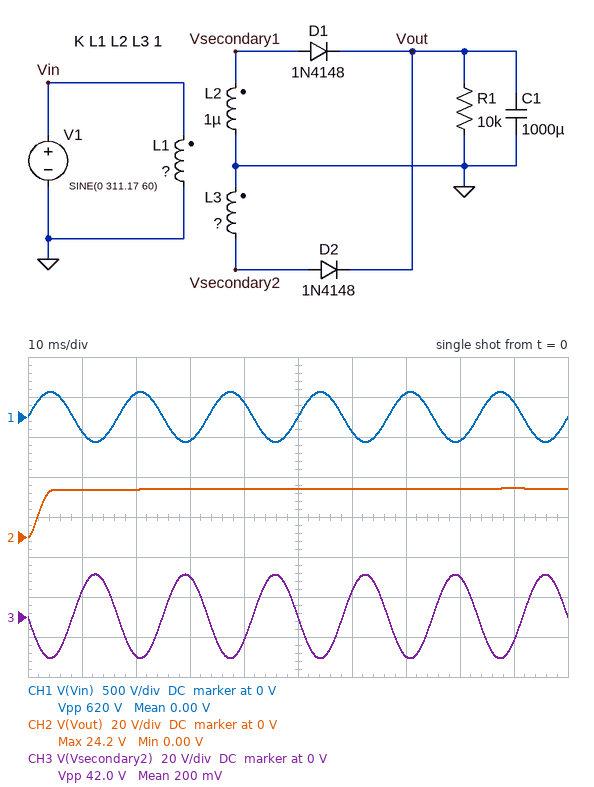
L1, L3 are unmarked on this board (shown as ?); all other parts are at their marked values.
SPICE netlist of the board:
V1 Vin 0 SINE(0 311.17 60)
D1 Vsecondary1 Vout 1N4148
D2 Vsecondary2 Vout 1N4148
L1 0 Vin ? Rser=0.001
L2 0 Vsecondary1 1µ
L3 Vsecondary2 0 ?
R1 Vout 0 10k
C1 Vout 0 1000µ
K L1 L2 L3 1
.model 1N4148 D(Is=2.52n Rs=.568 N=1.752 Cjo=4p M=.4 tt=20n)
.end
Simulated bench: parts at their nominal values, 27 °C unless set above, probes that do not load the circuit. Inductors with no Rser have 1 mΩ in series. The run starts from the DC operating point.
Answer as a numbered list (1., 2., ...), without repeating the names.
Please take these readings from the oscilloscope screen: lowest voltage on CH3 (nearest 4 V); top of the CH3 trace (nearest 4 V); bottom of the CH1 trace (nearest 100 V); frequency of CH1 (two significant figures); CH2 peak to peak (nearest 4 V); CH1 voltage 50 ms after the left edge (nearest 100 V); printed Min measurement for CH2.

1. -20 V
2. 20 V
3. -300 V
4. 60 Hz
5. 24 V
6. 0 V
7. 0.00 V
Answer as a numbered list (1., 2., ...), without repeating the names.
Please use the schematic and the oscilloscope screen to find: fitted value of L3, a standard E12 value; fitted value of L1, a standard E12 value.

1. 680 nH
2. 150 µH
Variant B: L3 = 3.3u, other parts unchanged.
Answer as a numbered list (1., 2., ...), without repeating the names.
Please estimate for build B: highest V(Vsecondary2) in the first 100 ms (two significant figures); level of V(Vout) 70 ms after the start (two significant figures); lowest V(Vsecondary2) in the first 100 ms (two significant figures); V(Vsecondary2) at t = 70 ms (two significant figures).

1. 47 V
2. 46 V
3. -46 V
4. -44 V
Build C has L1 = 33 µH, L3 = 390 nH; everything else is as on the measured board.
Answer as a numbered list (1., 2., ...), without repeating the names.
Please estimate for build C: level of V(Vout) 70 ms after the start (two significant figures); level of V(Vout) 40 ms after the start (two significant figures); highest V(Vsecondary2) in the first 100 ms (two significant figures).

1. 52 V
2. 51 V
3. 36 V
